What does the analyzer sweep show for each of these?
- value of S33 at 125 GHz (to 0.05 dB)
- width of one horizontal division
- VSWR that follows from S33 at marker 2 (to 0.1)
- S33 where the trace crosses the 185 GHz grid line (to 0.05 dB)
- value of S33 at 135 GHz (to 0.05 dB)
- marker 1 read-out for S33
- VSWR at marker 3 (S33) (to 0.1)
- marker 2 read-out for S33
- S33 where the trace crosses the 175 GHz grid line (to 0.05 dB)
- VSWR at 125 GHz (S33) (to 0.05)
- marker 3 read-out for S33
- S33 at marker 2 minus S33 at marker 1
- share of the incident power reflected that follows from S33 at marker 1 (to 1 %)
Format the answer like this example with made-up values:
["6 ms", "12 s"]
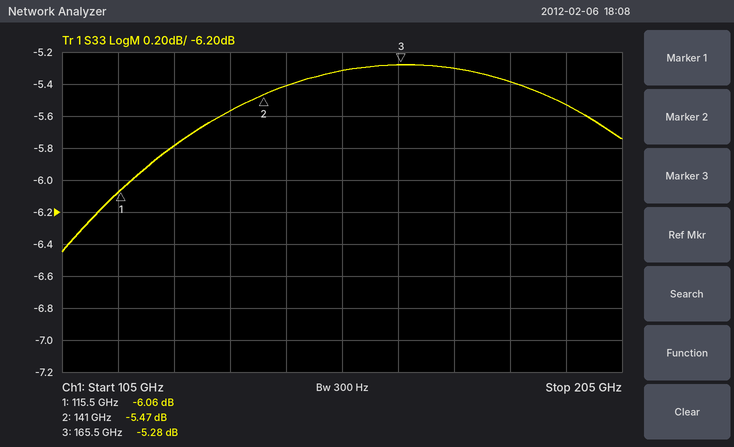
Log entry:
["-5.80 dB", "10 GHz", "3.3", "-5.40 dB", "-5.55 dB", "-6.06 dB", "3.4", "-5.47 dB", "-5.30 dB", "3.10", "-5.28 dB", "0.59 dB", "25 %"]
